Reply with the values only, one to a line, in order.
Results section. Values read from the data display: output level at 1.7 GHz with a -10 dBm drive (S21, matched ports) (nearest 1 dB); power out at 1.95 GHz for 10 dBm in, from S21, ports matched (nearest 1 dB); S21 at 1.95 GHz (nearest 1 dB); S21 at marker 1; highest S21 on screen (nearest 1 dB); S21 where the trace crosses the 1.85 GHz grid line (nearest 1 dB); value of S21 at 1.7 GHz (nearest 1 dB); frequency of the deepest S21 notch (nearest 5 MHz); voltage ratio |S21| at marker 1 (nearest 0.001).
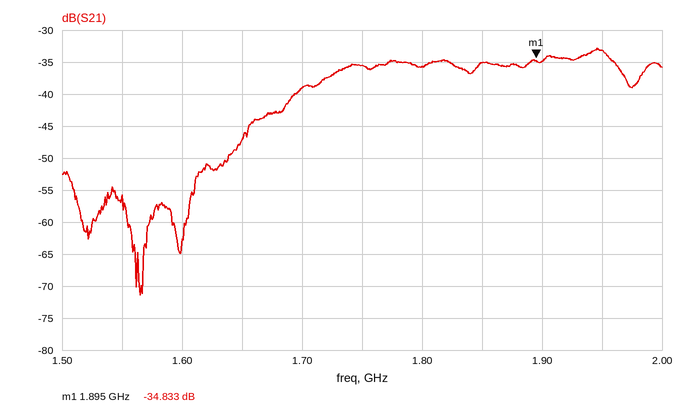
-49 dBm
-23 dBm
-33 dB
-34.833 dB
-33 dB
-35 dB
-39 dB
1.565 GHz
0.018
